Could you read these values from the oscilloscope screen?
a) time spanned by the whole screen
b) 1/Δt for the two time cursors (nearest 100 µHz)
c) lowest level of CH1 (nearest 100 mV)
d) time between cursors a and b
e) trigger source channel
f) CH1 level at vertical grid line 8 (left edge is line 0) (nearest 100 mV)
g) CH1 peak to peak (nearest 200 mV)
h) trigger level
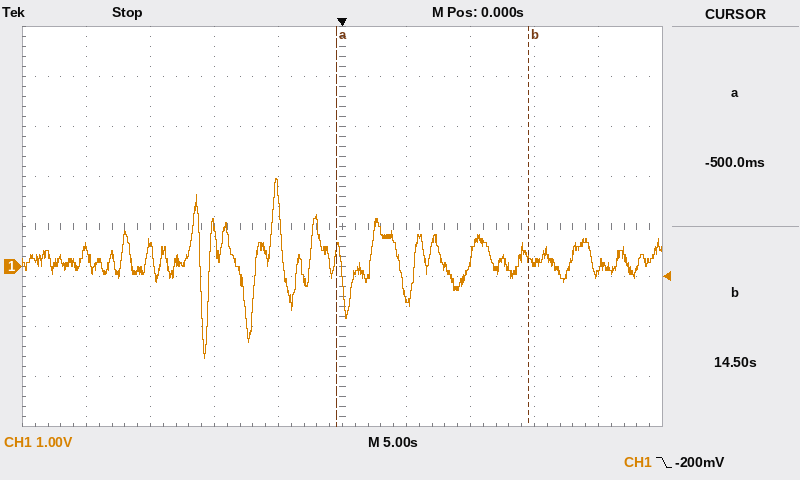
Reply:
50 s
66.7 mHz
-1.8 V
15.0 s
CH1
100 mV
3.6 V
-200 mV
